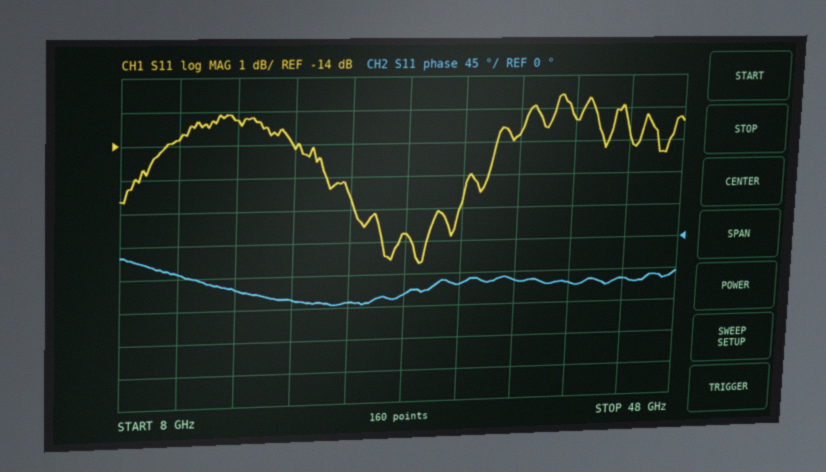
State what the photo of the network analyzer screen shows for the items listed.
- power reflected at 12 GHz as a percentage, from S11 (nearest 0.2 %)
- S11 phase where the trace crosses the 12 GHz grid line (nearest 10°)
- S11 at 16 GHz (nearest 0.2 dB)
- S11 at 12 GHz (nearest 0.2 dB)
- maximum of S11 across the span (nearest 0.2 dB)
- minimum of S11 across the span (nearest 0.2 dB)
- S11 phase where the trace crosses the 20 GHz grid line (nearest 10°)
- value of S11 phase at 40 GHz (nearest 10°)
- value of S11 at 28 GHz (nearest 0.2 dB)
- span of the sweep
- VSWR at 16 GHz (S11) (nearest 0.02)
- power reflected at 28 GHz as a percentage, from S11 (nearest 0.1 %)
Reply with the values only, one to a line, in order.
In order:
4.2 %
-40°
-13.2 dB
-13.8 dB
-12.6 dB
-17.6 dB
-80°
-60°
-16.8 dB
40 GHz
1.56
2.1 %
